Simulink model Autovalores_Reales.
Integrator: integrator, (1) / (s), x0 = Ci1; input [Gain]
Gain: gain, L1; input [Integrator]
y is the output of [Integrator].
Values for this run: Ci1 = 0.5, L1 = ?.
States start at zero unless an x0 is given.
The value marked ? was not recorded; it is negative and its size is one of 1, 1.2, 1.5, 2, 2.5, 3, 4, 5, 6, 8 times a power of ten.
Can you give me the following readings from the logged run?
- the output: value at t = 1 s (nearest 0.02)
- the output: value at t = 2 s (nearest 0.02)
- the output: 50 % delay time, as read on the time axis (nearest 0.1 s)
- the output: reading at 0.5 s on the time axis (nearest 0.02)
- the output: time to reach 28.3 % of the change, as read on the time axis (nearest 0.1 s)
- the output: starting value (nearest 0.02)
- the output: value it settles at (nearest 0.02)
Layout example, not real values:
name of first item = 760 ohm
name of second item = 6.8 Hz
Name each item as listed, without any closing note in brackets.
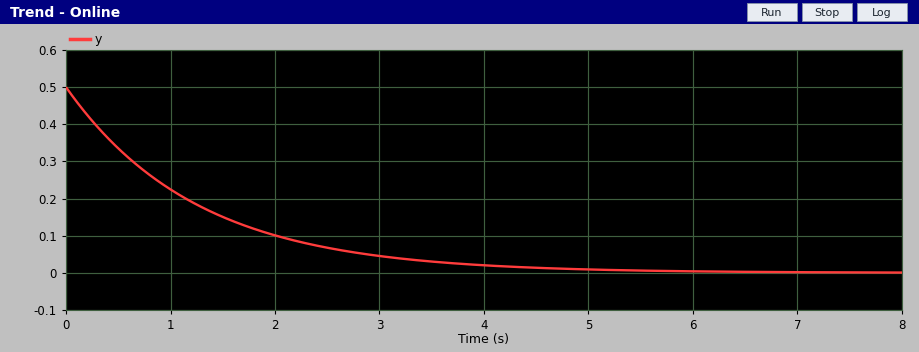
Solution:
the output: value at t = 1 s = 0.22
the output: value at t = 2 s = 0.10
the output: 50 % delay time, as read on the time axis = 0.9 s
the output: reading at 0.5 s on the time axis = 0.34
the output: time to reach 28.3 % of the change, as read on the time axis = 0.4 s
the output: starting value = 0.50
the output: value it settles at = 0.00
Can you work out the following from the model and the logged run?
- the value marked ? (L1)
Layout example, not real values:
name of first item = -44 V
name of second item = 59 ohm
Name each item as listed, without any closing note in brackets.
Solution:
the value marked ? = -0.8
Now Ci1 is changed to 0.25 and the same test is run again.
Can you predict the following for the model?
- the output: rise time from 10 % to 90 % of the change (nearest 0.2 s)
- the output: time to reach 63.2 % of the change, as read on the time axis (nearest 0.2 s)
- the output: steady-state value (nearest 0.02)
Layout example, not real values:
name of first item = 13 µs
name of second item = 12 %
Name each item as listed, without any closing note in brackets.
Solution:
the output: rise time from 10 % to 90 % of the change = 2.8 s
the output: time to reach 63.2 % of the change, as read on the time axis = 1.2 s
the output: steady-state value = 0.00
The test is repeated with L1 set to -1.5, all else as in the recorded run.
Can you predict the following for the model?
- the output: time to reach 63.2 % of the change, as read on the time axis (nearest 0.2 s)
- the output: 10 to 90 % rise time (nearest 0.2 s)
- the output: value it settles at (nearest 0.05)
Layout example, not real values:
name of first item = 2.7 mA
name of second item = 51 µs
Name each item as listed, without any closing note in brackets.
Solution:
the output: time to reach 63.2 % of the change, as read on the time axis = 0.6 s
the output: 10 to 90 % rise time = 1.4 s
the output: value it settles at = 0.00
